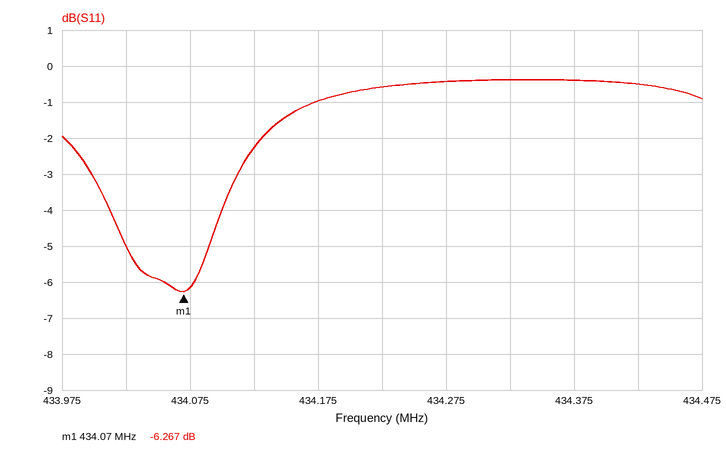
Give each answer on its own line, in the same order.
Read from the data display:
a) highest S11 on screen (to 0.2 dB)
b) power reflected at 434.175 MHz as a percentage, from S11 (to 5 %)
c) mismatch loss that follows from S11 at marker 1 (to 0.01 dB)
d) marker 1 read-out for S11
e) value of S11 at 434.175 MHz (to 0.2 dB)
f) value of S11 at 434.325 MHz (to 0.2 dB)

-0.4 dB
80 %
1.17 dB
-6.267 dB
-1.0 dB
-0.4 dB
